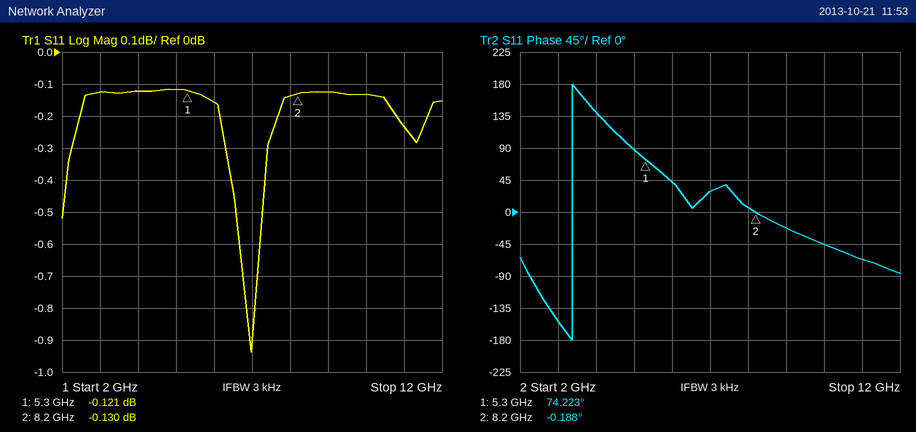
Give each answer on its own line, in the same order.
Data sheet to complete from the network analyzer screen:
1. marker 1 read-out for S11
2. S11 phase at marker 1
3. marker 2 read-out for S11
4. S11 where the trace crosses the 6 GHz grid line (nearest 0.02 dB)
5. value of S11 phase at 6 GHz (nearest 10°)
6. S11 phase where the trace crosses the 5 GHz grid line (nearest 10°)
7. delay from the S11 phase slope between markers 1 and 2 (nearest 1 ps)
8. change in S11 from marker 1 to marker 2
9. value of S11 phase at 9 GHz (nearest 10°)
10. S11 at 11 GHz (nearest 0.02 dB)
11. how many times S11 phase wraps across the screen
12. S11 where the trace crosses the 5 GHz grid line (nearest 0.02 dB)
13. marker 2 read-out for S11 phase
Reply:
-0.121 dB
74.223°
-0.130 dB
-0.16 dB
40°
90°
71 ps
-0.009 dB
-20°
-0.24 dB
1
-0.12 dB
-0.188°
